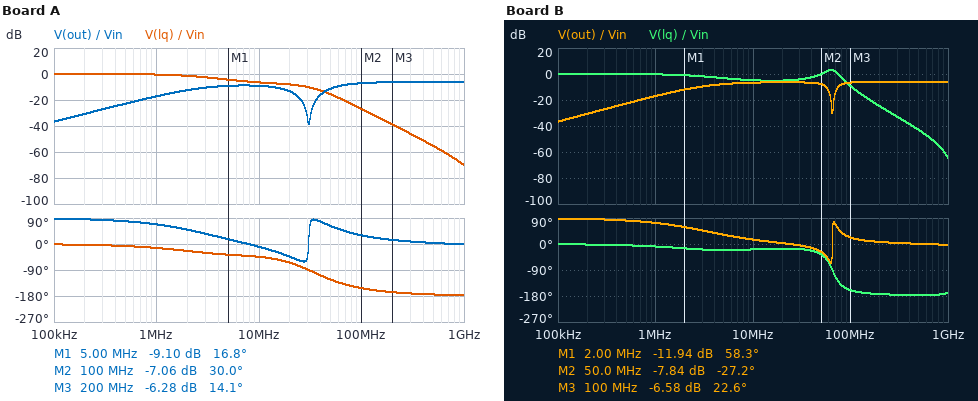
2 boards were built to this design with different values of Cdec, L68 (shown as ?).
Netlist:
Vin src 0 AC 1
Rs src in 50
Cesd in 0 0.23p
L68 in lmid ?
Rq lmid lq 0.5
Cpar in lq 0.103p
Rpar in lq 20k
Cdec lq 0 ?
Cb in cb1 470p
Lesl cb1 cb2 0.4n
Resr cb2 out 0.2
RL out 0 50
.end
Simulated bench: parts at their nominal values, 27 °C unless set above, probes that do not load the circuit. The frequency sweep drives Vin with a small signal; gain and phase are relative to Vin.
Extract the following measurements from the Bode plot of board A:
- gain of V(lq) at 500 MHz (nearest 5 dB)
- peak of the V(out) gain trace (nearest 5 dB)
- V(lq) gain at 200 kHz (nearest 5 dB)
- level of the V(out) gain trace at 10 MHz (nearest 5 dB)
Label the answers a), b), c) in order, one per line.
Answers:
a) -55 dB
b) -5 dB
c) 0 dB
d) -10 dB
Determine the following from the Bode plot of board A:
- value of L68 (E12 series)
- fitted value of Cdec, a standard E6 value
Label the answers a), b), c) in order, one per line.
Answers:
a) 82 nH
b) 330 pF
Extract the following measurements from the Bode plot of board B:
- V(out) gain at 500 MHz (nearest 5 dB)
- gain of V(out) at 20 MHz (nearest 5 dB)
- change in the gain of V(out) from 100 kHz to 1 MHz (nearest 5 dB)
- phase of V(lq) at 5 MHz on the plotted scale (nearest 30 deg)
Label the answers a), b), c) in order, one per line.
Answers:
a) -5 dB
b) -5 dB
c) 20 dB
d) -30 deg
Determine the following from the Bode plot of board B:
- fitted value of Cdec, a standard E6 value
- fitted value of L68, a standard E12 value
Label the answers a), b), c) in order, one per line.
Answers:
a) 33 pF
b) 180 nH
